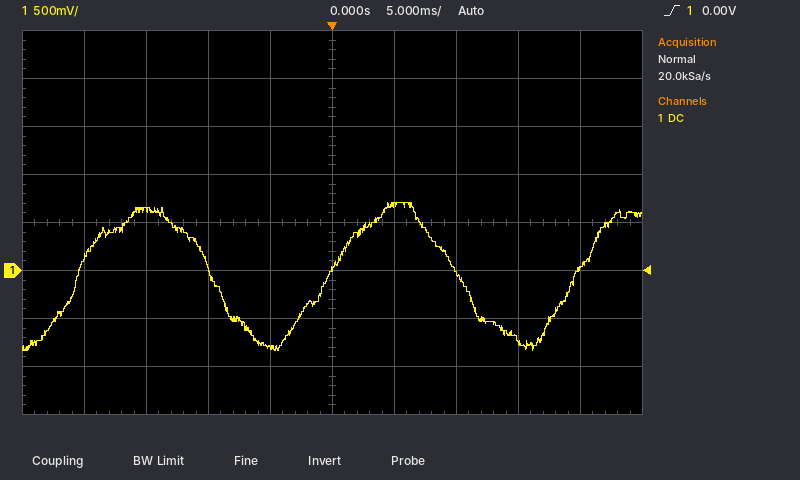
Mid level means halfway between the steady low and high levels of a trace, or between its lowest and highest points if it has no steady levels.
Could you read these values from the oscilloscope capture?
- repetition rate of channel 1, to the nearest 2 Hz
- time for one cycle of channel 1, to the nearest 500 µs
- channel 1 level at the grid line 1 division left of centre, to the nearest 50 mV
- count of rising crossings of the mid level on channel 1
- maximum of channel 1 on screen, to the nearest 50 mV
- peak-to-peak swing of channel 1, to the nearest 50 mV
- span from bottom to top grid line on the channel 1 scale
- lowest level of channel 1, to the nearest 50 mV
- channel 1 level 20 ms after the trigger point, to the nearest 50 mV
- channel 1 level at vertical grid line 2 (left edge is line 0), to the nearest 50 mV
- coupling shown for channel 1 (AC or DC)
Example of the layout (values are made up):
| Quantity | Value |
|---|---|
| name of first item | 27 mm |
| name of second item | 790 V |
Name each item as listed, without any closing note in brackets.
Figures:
| Quantity | Value |
|---|---|
| repetition rate of channel 1, to the nearest 2 Hz | 50 Hz |
| time for one cycle of channel 1, to the nearest 500 µs | 20.0 ms |
| channel 1 level at the grid line 1 division left of centre, to the nearest 50 mV | -800 mV |
| count of rising crossings of the mid level on channel 1 | 3 |
| maximum of channel 1 on screen, to the nearest 50 mV | 700 mV |
| peak-to-peak swing of channel 1, to the nearest 50 mV | 1.55 V |
| span from bottom to top grid line on the channel 1 scale | 4 V |
| lowest level of channel 1, to the nearest 50 mV | -850 mV |
| channel 1 level 20 ms after the trigger point, to the nearest 50 mV | 50 mV |
| channel 1 level at vertical grid line 2 (left edge is line 0), to the nearest 50 mV | 650 mV |
| coupling shown for channel 1 | DC |
